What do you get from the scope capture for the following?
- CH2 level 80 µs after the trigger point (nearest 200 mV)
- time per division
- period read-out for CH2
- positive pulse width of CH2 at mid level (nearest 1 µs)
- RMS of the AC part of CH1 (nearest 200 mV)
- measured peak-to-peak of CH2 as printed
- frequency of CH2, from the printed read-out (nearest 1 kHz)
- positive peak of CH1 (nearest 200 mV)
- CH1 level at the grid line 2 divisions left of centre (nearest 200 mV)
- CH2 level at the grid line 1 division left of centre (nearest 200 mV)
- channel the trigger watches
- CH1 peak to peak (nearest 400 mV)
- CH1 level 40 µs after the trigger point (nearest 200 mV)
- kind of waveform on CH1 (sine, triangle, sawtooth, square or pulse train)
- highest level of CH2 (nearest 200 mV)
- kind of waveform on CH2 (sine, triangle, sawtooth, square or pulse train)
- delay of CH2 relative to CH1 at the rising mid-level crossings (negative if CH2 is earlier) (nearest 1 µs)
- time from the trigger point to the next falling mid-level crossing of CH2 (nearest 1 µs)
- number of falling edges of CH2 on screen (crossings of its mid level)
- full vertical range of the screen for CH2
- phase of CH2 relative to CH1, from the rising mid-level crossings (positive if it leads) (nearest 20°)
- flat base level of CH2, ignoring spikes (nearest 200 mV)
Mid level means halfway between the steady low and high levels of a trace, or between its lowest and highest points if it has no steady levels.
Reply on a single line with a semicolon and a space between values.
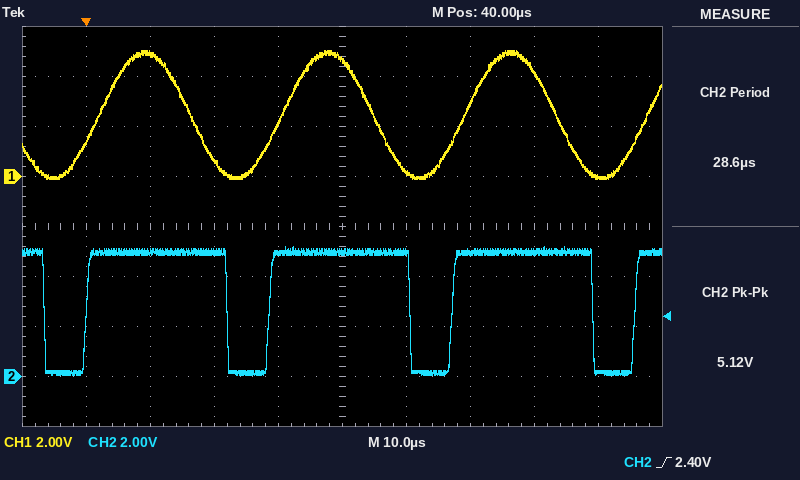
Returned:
200 mV; 10 µs; 28.6 µs; 22 µs; 1.8 V; 5.12 V; 35 kHz; 5.0 V; 600 mV; 5.0 V; CH2; 5.2 V; 4.6 V; sine; 5.2 V; pulse train; -2 µs; 22 µs; 4; 16 V; +20°; 200 mV
